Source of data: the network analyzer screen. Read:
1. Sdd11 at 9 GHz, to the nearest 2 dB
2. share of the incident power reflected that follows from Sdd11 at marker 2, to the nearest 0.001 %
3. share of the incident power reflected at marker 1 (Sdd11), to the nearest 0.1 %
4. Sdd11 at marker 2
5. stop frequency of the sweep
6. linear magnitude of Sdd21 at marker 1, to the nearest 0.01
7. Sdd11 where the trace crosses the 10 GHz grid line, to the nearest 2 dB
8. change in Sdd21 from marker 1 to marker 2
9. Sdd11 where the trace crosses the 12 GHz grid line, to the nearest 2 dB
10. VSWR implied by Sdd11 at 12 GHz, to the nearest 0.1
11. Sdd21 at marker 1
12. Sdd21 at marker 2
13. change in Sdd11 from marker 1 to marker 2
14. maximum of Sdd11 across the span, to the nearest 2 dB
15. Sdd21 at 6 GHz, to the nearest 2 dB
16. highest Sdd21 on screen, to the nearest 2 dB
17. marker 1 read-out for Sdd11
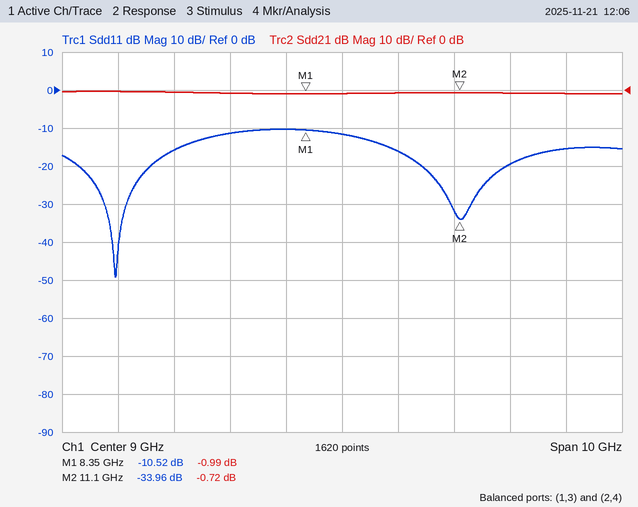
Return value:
-12 dB
0.040 %
8.9 %
-33.96 dB
14 GHz
0.89
-16 dB
0.27 dB
-20 dB
1.2
-0.99 dB
-0.72 dB
-23.44 dB
-10 dB
0 dB
0 dB
-10.52 dB
